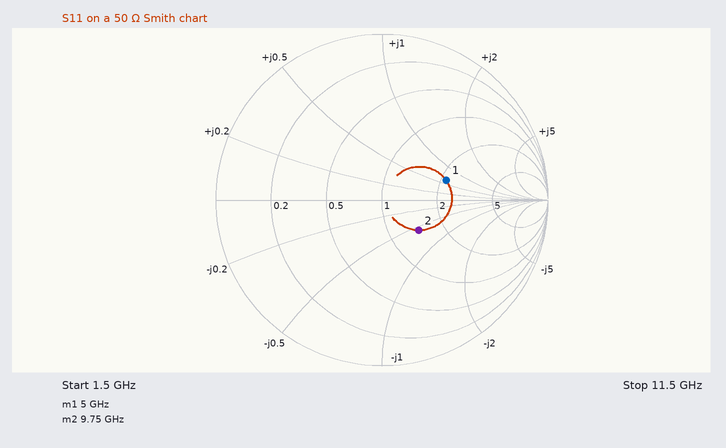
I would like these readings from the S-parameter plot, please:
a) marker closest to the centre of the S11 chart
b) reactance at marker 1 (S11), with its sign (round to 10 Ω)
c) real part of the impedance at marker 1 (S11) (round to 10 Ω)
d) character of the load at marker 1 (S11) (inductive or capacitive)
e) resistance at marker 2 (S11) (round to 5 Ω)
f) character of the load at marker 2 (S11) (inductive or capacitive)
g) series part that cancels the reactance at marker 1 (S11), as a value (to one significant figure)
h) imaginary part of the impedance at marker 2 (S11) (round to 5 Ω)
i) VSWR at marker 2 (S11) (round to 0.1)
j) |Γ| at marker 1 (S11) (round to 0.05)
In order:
marker 2
+30 Ω
110 Ω
inductive
70 Ω
capacitive
1 pF
-30 Ω
1.8
0.40
